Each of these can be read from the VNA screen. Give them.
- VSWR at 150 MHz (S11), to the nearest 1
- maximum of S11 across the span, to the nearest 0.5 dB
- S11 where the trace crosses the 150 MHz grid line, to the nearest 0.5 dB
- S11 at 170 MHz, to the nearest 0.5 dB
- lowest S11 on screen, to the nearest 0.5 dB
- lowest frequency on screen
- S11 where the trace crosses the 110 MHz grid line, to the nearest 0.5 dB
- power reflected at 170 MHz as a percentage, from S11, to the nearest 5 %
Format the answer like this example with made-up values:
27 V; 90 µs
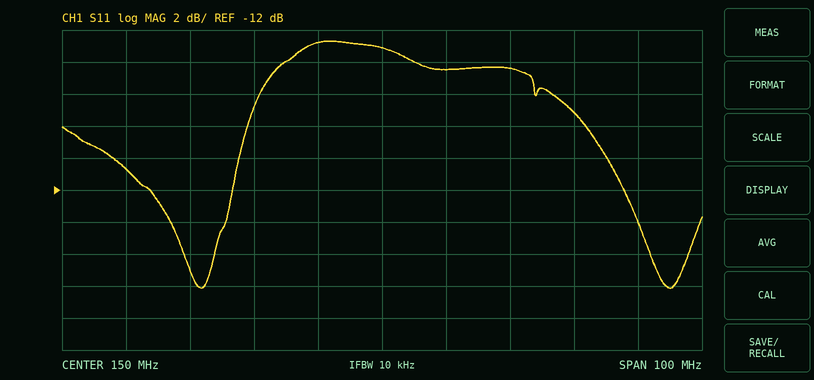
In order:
6; -2.5 dB; -3.0 dB; -4.5 dB; -18.0 dB; 100 MHz; -10.5 dB; 35 %
